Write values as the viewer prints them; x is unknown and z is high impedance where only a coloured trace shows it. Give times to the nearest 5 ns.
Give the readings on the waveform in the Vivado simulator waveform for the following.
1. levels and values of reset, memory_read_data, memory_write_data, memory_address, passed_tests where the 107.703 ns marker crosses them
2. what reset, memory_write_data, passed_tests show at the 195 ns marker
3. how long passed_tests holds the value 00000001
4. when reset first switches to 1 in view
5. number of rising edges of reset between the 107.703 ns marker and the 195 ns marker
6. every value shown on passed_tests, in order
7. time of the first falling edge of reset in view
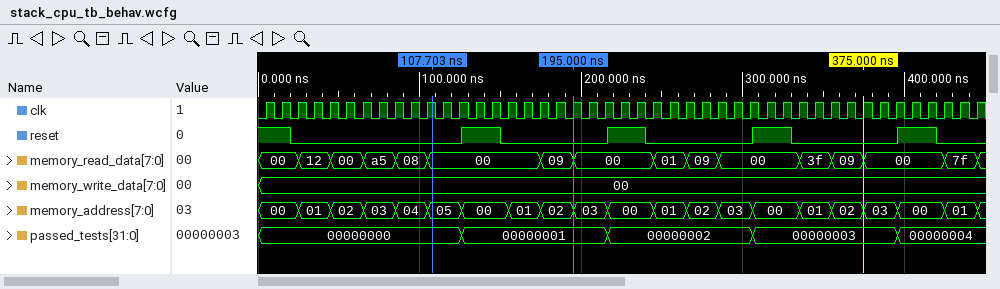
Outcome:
reset=0, memory_read_data=00, memory_write_data=00, memory_address=05, passed_tests=00000000
reset=0, memory_write_data=00, passed_tests=00000001
90 ns
125 ns
1
00000000, 00000001, 00000002, 00000003, 00000004
20 ns
